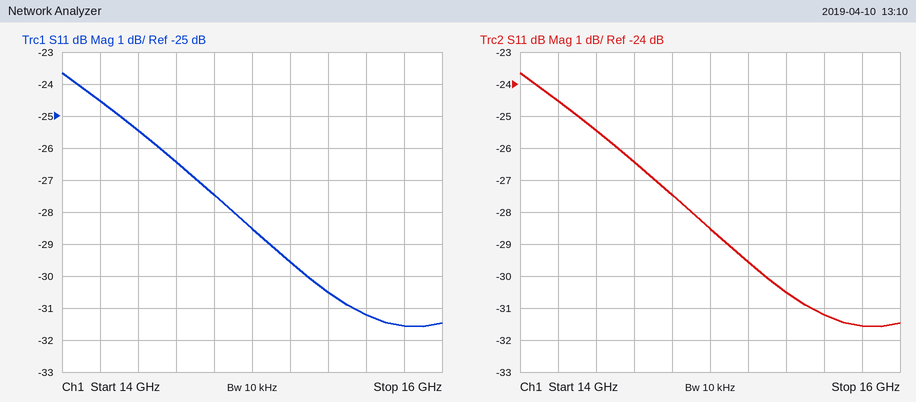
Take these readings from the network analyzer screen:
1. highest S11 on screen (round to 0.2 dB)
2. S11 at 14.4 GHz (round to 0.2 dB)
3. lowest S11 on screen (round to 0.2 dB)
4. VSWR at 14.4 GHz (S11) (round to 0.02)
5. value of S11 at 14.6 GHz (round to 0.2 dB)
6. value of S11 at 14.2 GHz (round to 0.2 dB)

-23.6 dB
-25.4 dB
-31.6 dB
1.12
-26.4 dB
-24.6 dB
